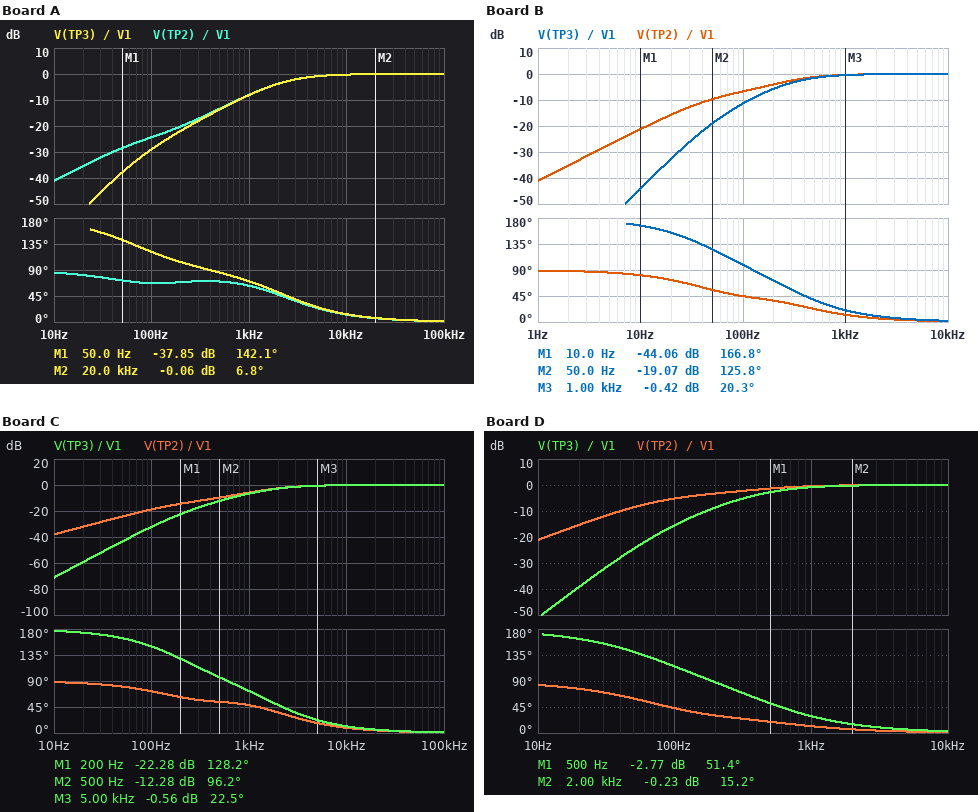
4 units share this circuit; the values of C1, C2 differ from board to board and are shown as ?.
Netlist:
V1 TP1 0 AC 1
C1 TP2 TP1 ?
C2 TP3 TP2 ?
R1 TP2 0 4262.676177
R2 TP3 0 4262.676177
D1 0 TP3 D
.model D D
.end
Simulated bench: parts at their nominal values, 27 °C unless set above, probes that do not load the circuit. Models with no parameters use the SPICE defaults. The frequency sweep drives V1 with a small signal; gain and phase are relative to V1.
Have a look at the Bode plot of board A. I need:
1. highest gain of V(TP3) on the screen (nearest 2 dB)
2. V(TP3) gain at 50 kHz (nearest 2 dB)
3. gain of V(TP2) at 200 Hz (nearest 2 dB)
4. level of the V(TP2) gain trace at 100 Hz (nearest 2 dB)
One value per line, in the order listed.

0 dB
0 dB
-20 dB
-24 dB
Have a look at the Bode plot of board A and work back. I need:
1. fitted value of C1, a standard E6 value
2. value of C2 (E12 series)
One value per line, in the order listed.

33 nF
270 nF
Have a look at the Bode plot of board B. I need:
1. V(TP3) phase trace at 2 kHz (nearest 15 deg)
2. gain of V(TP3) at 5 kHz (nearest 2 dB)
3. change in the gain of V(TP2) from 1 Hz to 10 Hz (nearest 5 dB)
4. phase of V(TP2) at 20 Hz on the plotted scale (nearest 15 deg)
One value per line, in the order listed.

15 deg
0 dB
20 dB
75 deg
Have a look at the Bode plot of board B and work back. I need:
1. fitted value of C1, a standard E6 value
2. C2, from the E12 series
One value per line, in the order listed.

330 nF
270 nF
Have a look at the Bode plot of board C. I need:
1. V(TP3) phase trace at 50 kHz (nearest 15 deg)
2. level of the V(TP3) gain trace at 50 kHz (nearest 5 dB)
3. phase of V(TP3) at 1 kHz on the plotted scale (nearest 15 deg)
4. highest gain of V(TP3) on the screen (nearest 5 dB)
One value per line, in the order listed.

0 deg
0 dB
75 deg
0 dB
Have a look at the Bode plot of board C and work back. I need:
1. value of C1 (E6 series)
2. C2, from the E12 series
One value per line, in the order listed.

47 nF
82 nF
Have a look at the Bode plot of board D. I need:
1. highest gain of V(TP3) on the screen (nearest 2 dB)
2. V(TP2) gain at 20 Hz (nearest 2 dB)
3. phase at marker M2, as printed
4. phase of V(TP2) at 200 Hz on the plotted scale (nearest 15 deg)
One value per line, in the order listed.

0 dB
-16 dB
15.2 deg
30 deg
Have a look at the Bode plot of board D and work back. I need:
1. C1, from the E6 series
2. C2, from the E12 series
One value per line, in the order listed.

330 nF
120 nF
